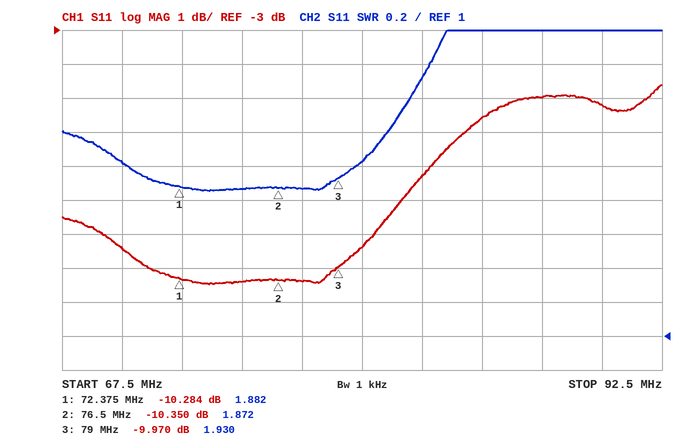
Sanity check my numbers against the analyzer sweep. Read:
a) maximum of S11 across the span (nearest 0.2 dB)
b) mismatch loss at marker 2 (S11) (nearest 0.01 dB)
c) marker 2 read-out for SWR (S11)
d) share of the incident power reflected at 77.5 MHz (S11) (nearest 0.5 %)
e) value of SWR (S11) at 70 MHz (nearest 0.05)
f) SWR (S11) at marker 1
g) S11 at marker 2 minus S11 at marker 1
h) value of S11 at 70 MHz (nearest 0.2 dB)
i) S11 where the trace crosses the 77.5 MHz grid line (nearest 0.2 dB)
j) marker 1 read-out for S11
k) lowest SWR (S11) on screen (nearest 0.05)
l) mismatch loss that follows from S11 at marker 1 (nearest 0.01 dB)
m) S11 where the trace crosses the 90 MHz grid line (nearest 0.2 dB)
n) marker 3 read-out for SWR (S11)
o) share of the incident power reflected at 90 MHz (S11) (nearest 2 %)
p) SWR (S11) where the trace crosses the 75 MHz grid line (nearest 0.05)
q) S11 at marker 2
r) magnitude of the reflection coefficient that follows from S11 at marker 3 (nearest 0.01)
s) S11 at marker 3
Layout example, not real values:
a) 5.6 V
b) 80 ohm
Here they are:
a) -4.6 dB
b) 0.42 dB
c) 1.872
d) 9.0 %
e) 2.00
f) 1.882
g) -0.066 dB
h) -9.4 dB
i) -10.4 dB
j) -10.284 dB
k) 1.85
l) 0.43 dB
m) -5.2 dB
n) 1.930
o) 30 %
p) 1.85
q) -10.350 dB
r) 0.32
s) -9.970 dB
